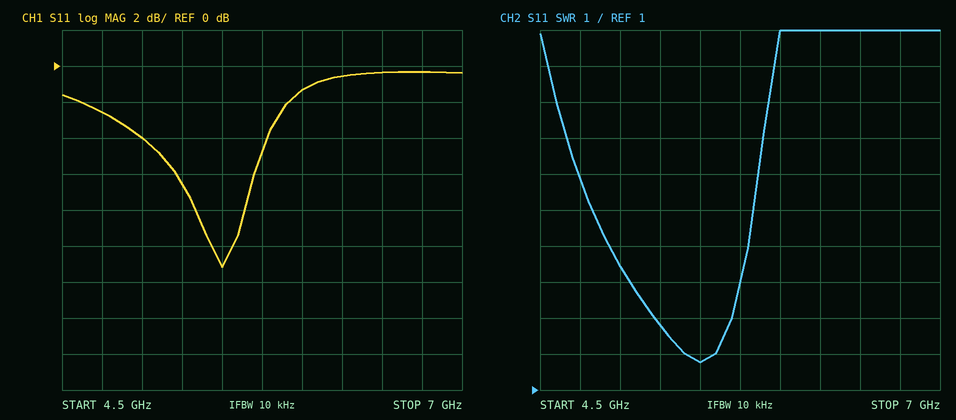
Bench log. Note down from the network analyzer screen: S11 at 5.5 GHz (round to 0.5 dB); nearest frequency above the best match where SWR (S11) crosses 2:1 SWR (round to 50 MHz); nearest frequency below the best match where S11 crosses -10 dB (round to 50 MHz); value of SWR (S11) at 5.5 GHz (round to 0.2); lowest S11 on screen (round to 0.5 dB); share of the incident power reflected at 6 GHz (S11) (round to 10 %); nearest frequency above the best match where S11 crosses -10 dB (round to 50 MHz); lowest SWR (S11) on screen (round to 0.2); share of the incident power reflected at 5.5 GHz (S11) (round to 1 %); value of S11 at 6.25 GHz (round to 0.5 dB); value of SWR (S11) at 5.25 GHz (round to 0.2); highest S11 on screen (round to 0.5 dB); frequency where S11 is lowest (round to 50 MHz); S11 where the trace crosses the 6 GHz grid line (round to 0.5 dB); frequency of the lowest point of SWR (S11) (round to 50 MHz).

-11.0 dB
5.60 GHz
5.45 GHz
1.8
-11.0 dB
70 %
5.55 GHz
1.8
8 %
-0.5 dB
2.8
-0.5 dB
5.50 GHz
-1.5 dB
5.50 GHz
